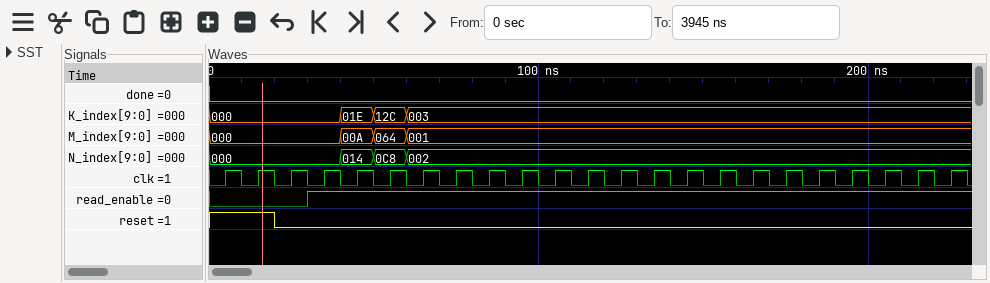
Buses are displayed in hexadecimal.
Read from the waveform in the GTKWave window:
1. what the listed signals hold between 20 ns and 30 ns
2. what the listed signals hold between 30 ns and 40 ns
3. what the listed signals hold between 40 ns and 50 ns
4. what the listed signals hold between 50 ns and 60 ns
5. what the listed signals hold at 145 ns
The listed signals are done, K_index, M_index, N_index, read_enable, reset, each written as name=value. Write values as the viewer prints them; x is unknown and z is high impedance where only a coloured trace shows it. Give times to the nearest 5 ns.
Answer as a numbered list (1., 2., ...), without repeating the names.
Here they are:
1. done=0, K_index=000, M_index=000, N_index=000, read_enable=0, reset=0
2. done=0, K_index=000, M_index=000, N_index=000, read_enable=1, reset=0
3. done=0, K_index=01E, M_index=00A, N_index=014, read_enable=1, reset=0
4. done=0, K_index=12C, M_index=064, N_index=0C8, read_enable=1, reset=0
5. done=0, K_index=003, M_index=001, N_index=002, read_enable=1, reset=0
